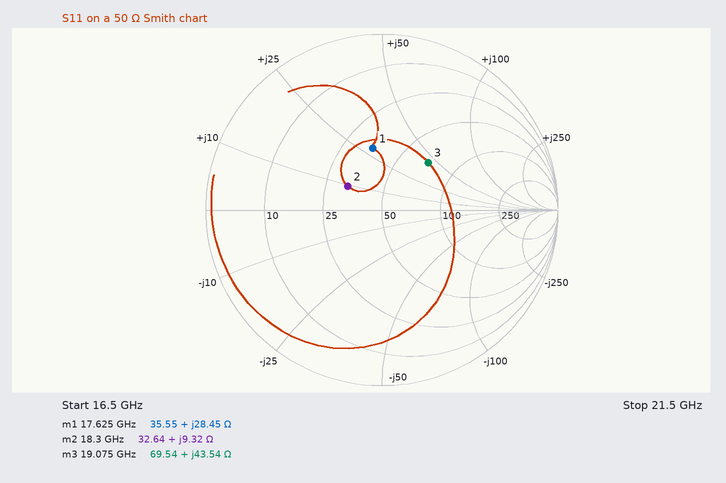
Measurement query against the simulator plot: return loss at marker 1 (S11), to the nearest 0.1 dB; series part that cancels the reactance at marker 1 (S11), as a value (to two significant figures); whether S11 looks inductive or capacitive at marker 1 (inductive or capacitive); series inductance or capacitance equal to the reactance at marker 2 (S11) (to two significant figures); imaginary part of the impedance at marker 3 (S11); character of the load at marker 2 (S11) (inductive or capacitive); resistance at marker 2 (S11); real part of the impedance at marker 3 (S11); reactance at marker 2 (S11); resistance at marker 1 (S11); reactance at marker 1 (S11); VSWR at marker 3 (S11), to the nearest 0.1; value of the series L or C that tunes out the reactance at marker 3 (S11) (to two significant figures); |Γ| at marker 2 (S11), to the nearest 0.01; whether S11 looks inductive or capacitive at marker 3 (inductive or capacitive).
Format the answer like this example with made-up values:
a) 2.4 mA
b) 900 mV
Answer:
a) 9.0 dB
b) 320 fF
c) inductive
d) 81 pH
e) +43.54 Ω
f) inductive
g) 32.64 Ω
h) 69.54 Ω
i) +9.32 Ω
j) 35.55 Ω
k) +28.45 Ω
l) 2.2
m) 190 fF
n) 0.24
o) inductive
